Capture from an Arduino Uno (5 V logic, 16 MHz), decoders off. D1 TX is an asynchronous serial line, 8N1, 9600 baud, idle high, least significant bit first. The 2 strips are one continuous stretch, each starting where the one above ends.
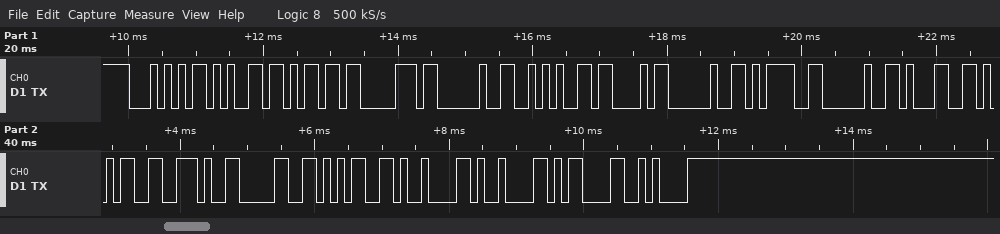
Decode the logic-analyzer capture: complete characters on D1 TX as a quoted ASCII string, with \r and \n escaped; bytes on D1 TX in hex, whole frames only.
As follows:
"Temp *C = 15.05\t\t\r\n"
54 65 6D 70 20 2A 43 20 3D 20 31 35 2E 30 35 09 09 0D 0A
